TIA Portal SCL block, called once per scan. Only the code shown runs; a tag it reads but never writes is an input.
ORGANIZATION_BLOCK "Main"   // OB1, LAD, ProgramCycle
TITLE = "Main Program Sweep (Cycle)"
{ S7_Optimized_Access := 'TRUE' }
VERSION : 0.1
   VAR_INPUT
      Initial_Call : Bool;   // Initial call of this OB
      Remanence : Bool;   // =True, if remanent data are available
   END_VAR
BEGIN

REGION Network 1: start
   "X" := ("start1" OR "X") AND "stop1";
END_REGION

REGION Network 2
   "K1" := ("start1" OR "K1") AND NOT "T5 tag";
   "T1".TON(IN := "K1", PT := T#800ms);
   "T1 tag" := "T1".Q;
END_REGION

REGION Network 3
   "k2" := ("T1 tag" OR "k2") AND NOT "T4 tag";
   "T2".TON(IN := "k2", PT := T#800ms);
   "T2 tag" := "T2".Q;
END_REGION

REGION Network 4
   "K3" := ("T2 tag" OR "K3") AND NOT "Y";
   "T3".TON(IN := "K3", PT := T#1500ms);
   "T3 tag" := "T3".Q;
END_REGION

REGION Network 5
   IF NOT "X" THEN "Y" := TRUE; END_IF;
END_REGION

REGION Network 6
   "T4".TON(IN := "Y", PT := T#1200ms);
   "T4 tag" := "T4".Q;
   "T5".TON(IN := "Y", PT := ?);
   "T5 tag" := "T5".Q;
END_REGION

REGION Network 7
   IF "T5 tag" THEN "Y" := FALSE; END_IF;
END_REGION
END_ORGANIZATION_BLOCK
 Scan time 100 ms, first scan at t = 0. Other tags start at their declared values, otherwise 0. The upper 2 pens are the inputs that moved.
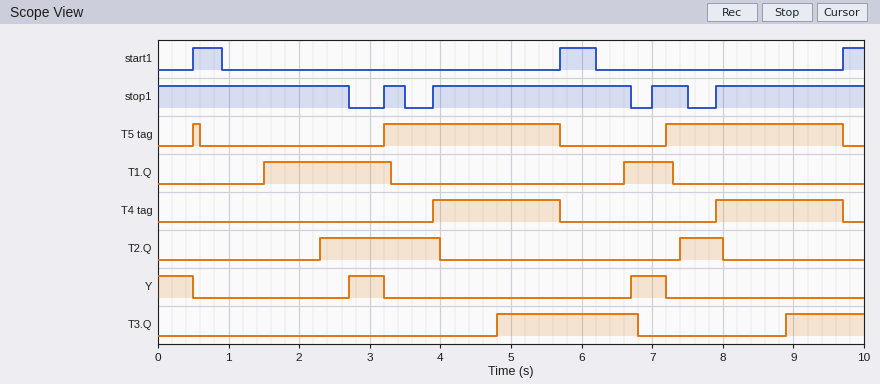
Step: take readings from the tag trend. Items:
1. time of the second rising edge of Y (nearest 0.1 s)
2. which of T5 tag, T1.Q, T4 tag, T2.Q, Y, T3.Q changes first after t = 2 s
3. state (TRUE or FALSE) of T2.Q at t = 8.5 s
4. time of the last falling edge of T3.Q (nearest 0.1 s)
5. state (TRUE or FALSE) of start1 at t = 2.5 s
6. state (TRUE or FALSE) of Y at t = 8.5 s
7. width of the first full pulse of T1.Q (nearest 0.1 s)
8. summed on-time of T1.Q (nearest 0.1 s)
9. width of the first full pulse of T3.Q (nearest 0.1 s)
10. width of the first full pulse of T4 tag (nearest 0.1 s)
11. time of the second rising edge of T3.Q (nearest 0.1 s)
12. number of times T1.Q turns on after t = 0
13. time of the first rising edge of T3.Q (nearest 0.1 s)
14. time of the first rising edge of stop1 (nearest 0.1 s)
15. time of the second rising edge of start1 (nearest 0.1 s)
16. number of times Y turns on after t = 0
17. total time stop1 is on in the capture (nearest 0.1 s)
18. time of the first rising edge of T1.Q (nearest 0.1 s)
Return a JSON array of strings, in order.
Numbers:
["6.7 s", "T2.Q", "FALSE", "6.8 s", "FALSE", "FALSE", "1.8 s", "2.5 s", "2.0 s", "1.8 s", "8.9 s", "2", "4.8 s", "3.2 s", "5.7 s", "2", "8.4 s", "1.5 s"]
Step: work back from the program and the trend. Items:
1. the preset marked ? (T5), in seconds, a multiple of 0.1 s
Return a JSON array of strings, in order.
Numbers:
["0.5 s"]
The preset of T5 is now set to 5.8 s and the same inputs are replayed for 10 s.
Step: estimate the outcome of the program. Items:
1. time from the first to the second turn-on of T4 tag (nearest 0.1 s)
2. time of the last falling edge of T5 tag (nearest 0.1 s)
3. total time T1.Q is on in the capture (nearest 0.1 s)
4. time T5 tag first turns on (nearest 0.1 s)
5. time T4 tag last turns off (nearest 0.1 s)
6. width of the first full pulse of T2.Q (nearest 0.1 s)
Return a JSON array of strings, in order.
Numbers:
["6.7 s", "5.9 s", "7.8 s", "5.8 s", "5.9 s", "0.4 s"]
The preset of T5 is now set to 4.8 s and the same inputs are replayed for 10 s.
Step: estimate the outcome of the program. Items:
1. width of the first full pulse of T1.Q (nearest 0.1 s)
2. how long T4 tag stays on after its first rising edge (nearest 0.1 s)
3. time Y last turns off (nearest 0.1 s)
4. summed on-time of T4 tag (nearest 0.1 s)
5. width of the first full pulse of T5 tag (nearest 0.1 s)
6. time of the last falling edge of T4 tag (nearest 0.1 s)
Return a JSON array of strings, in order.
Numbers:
["3.6 s", "4.5 s", "4.8 s", "6.6 s", "0.9 s", "5.7 s"]
